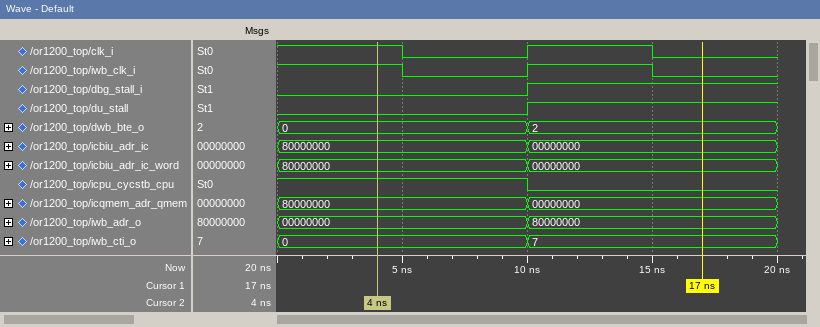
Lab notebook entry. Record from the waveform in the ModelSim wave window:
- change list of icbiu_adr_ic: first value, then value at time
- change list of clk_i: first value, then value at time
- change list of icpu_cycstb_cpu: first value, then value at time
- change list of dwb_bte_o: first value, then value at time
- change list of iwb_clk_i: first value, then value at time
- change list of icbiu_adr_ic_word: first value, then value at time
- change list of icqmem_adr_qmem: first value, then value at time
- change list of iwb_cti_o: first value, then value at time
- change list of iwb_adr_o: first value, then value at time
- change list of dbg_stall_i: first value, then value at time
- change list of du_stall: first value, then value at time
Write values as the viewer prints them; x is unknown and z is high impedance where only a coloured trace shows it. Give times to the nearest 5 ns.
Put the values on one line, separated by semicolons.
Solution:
80000000, 00000000 at 10 ns; 1, 0 at 5 ns, 1 at 10 ns, 0 at 15 ns; 1, 0 at 10 ns; 0, 2 at 10 ns; 1, 0 at 5 ns, 1 at 10 ns, 0 at 15 ns; 80000000, 00000000 at 10 ns; 80000000, 00000000 at 10 ns; 0, 7 at 10 ns; 00000000, 80000000 at 10 ns; 0, 1 at 10 ns; 0, 1 at 10 ns
